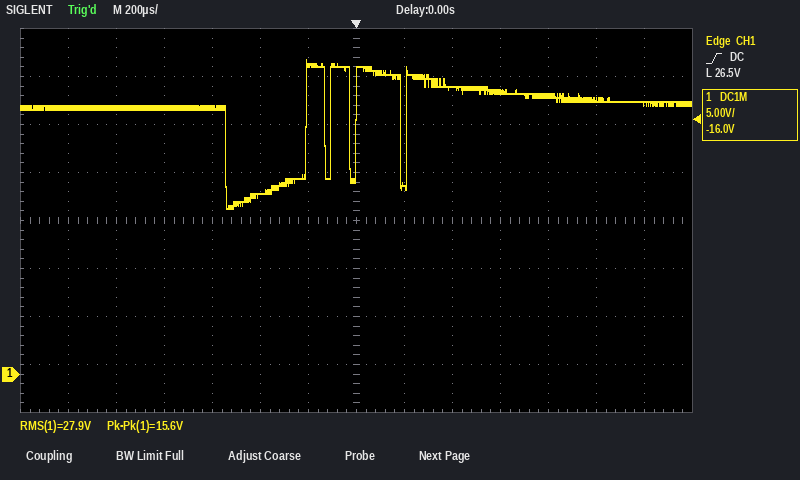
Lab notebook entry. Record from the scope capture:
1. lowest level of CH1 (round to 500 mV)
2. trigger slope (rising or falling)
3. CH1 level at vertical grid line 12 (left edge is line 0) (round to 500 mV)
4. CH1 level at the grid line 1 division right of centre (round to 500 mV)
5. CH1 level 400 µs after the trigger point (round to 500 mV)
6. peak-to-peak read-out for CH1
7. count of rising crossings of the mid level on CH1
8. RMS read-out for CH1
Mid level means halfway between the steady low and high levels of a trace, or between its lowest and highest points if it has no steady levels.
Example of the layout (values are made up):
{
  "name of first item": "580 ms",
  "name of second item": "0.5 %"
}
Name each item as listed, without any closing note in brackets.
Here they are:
{
  "lowest level of CH1": "17.0 V",
  "trigger slope": "rising",
  "CH1 level at vertical grid line 12 (left edge is line 0)": "28.5 V",
  "CH1 level at the grid line 1 division right of centre": "19.5 V",
  "CH1 level 400 µs after the trigger point": "30.0 V",
  "peak-to-peak read-out for CH1": "15.6 V",
  "count of rising crossings of the mid level on CH1": "4",
  "RMS read-out for CH1": "27.9 V"
}
